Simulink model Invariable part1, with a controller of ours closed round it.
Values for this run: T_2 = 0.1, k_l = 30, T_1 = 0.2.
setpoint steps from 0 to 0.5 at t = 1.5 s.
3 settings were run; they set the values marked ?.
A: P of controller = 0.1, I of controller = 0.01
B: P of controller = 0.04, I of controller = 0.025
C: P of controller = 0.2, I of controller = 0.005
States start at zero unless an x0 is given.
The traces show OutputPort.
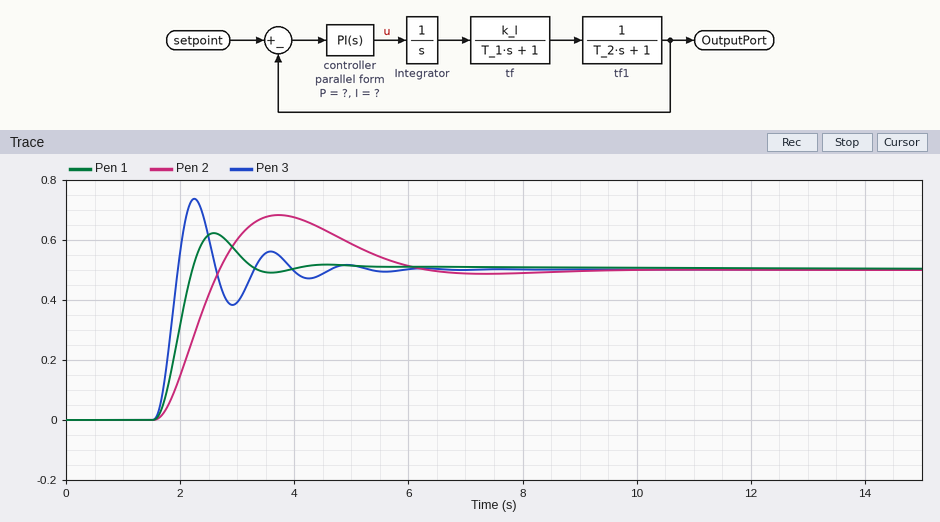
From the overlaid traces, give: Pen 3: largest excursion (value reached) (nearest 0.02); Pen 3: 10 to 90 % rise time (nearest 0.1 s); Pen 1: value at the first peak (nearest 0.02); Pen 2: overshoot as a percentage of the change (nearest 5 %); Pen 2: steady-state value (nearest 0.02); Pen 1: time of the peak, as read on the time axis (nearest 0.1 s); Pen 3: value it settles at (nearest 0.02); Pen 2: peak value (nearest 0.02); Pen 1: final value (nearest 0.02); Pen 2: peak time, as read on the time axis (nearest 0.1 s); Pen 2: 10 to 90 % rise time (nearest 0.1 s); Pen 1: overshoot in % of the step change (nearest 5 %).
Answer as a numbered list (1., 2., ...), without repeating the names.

1. 0.74
2. 0.3 s
3. 0.62
4. 35 %
5. 0.50
6. 2.6 s
7. 0.50
8. 0.68
9. 0.50
10. 3.7 s
11. 0.8 s
12. 25 %
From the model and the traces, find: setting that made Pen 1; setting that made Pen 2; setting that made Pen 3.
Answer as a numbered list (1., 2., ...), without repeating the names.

1. A
2. B
3. C
